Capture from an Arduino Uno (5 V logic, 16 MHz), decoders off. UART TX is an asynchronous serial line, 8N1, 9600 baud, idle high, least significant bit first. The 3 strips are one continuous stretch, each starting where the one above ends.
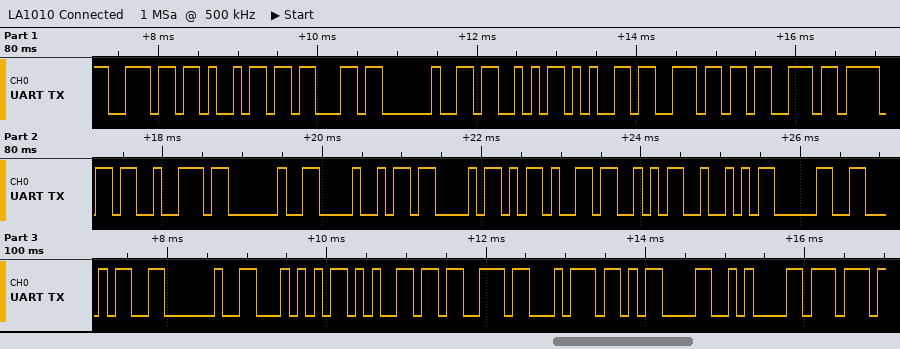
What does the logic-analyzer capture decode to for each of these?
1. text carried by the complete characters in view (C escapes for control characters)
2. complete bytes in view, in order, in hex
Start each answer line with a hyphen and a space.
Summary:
- "nic Sensor HC-SR04 Test\r\nw"
- 6E 69 63 20 53 65 6E 73 6F 72 20 48 43 2D 53 52 30 34 20 54 65 73 74 0D 0A 77
